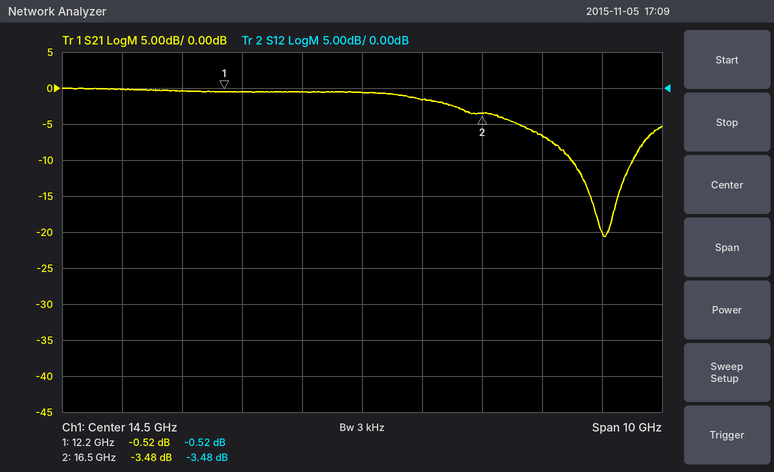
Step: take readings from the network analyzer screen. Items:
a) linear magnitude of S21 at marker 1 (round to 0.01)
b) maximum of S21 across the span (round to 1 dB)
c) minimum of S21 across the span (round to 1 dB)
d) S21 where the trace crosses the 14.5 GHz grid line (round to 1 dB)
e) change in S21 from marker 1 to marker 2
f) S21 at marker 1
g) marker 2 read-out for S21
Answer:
0.94
0 dB
-21 dB
-1 dB
-2.96 dB
-0.52 dB
-3.48 dB
